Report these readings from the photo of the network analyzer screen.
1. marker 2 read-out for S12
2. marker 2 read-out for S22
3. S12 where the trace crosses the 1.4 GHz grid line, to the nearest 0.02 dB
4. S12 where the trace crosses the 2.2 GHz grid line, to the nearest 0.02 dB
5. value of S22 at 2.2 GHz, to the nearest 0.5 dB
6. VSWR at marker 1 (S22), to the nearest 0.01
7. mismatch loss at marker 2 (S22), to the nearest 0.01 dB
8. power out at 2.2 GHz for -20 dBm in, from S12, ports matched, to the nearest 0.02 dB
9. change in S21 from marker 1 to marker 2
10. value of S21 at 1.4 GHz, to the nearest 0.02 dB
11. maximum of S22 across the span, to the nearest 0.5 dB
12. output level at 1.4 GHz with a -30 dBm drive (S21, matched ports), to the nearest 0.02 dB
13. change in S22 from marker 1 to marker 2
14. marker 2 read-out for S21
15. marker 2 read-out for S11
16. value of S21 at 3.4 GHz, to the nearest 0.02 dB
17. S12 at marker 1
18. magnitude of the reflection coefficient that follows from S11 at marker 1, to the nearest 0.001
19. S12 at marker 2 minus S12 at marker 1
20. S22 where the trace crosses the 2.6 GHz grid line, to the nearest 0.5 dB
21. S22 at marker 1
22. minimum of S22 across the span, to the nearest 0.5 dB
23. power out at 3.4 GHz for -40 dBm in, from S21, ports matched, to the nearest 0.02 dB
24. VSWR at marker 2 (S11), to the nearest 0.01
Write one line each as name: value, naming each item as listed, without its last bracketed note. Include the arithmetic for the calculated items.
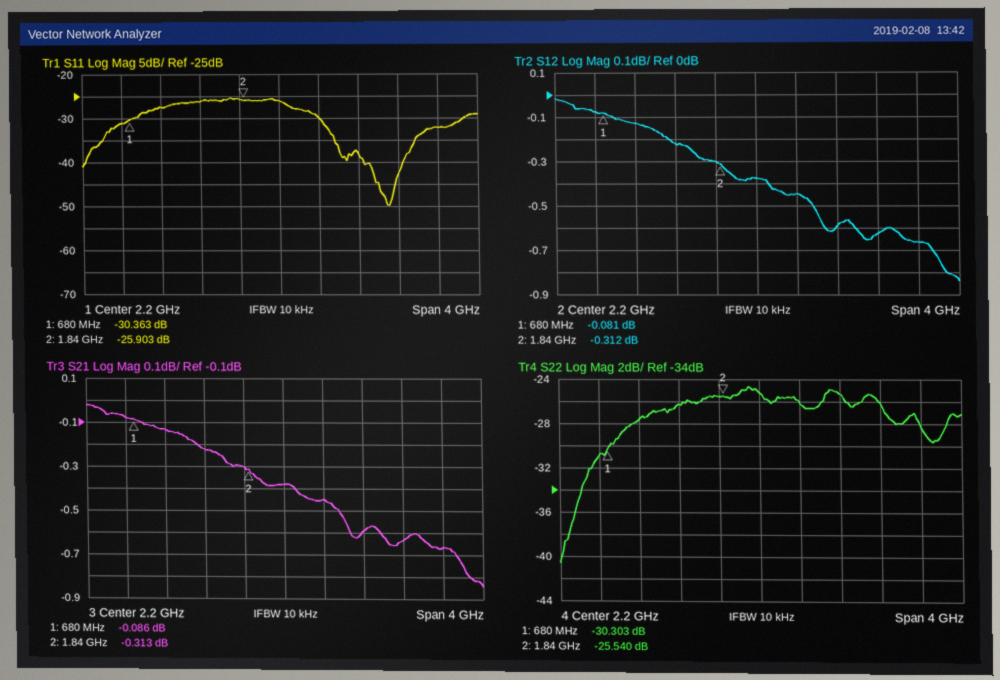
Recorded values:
marker 2 read-out for S12: -0.312 dB
marker 2 read-out for S22: -25.540 dB
S12 where the trace crosses the 1.4 GHz grid line, to the nearest 0.02 dB: -0.22 dB
S12 where the trace crosses the 2.2 GHz grid line, to the nearest 0.02 dB: -0.38 dB
value of S22 at 2.2 GHz, to the nearest 0.5 dB: -25.0 dB
VSWR at marker 1 (S22), to the nearest 0.01: (1 + 0.0305)/(1 − 0.0305) ≈ 1.06
mismatch loss at marker 2 (S22), to the nearest 0.01 dB: −10 log10(1 − 10^(-25.54/10)) ≈ 0.01 dB
power out at 2.2 GHz for -20 dBm in, from S12, ports matched, to the nearest 0.02 dB: -20 dBm + (-0.38 dB) = -20.38 dBm
change in S21 from marker 1 to marker 2: -0.313 − (-0.086) = -0.227 dB
value of S21 at 1.4 GHz, to the nearest 0.02 dB: -0.22 dB
maximum of S22 across the span, to the nearest 0.5 dB: -24.5 dB
output level at 1.4 GHz with a -30 dBm drive (S21, matched ports), to the nearest 0.02 dB: -30 dBm + (-0.22 dB) = -30.22 dBm
change in S22 from marker 1 to marker 2: -25.54 − (-30.303) = 4.763 dB
marker 2 read-out for S21: -0.313 dB
marker 2 read-out for S11: -25.903 dB
value of S21 at 3.4 GHz, to the nearest 0.02 dB: -0.64 dB
S12 at marker 1: -0.081 dB
magnitude of the reflection coefficient that follows from S11 at marker 1, to the nearest 0.001: 10^(-30.363/20) ≈ 0.030
S12 at marker 2 minus S12 at marker 1: -0.312 − (-0.081) = -0.231 dB
S22 where the trace crosses the 2.6 GHz grid line, to the nearest 0.5 dB: -26.0 dB
S22 at marker 1: -30.303 dB
minimum of S22 across the span, to the nearest 0.5 dB: -40.5 dB
power out at 3.4 GHz for -40 dBm in, from S21, ports matched, to the nearest 0.02 dB: -40 dBm + (-0.64 dB) = -40.64 dBm
VSWR at marker 2 (S11), to the nearest 0.01: (1 + 0.0507)/(1 − 0.0507) ≈ 1.11
